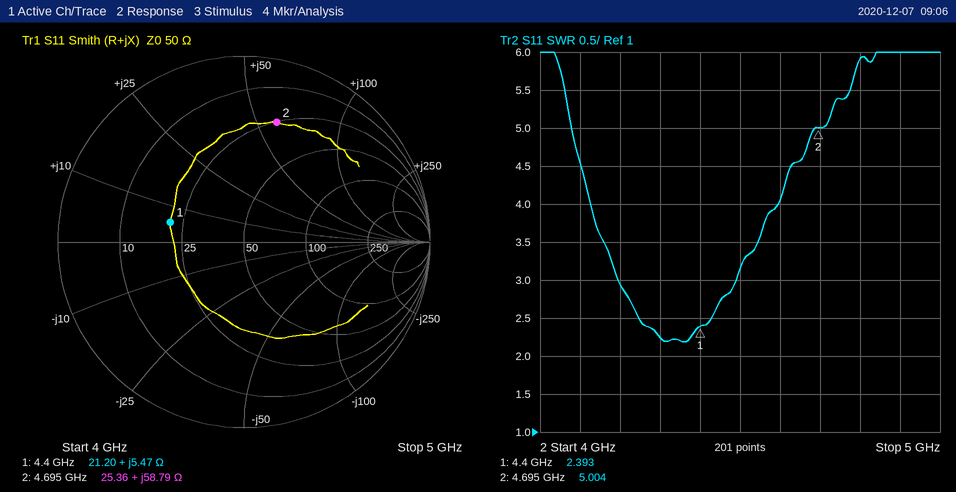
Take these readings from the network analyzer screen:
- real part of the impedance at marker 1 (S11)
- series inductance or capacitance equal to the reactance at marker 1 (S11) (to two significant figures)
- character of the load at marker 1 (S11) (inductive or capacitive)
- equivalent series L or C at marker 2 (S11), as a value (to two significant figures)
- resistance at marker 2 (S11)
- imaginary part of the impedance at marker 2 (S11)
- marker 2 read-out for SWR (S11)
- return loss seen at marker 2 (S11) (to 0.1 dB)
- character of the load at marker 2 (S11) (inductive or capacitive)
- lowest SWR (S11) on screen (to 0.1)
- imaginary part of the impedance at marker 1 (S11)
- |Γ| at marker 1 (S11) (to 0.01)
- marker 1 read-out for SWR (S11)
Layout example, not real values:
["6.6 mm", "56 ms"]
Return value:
["21.20 Ω", "200 pH", "inductive", "2.0 nH", "25.36 Ω", "+58.79 Ω", "5.004", "3.5 dB", "inductive", "2.2", "+5.47 Ω", "0.41", "2.393"]
